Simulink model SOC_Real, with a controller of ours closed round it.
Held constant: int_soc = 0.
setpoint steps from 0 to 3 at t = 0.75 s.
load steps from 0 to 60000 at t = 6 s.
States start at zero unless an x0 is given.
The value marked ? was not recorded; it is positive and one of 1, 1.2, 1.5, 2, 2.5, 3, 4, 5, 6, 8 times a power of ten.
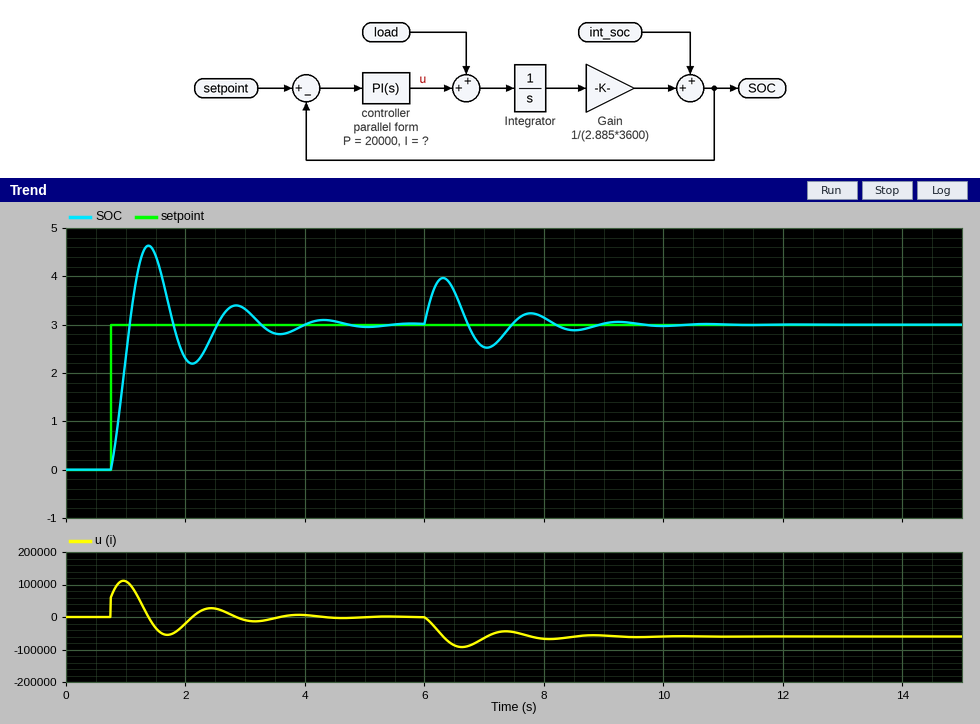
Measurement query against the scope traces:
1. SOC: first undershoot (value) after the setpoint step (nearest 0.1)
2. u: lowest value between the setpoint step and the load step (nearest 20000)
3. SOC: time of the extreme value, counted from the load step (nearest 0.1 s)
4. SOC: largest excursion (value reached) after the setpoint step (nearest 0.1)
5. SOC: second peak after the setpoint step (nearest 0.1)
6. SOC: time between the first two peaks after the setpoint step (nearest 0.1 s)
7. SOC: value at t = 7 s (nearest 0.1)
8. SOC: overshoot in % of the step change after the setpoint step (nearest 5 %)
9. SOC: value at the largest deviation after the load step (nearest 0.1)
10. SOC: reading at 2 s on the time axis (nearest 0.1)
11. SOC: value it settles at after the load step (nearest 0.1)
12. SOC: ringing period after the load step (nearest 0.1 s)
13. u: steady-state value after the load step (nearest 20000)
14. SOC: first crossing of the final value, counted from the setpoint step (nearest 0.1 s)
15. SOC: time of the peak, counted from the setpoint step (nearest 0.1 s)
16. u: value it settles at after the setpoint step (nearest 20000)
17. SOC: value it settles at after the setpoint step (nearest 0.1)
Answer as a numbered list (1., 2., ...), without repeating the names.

1. 2.2
2. -60000
3. 0.3 s
4. 4.6
5. 3.4
6. 1.5 s
7. 2.5
8. 55 %
9. 4.0
10. 2.3
11. 3.0
12. 1.5 s
13. -60000
14. 0.3 s
15. 0.6 s
16. 0
17. 3.0
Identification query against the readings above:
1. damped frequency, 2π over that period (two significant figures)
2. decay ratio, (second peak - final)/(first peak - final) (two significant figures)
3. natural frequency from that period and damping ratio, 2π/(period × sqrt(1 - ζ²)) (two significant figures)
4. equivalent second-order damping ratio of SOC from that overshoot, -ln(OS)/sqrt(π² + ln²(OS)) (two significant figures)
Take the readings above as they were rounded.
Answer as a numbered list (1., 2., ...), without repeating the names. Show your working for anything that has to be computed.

1. 2π / 1.5 = 4.2 rad/s
2. (3.4 - 3) / (4.6 - 3) = 0.25
3. 2π / (1.5 × sqrt(1 - 0.19²)) = 4.3 rad/s
4. ln(0.55) = -0.598; 0.598 / sqrt(9.870 + 0.357) = 0.19
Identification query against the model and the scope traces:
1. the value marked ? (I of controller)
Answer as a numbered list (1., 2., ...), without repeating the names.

1. 200000
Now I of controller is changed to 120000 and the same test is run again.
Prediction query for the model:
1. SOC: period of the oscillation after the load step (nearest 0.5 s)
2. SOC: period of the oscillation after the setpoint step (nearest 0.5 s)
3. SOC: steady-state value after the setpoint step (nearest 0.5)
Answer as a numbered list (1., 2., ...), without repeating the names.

1. 2.0 s
2. 2.0 s
3. 3.0
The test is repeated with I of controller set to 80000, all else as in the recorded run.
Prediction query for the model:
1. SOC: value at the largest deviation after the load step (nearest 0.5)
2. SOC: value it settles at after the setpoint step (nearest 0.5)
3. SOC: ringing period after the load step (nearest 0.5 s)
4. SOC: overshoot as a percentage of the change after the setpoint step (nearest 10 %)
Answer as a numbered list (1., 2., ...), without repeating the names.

1. 4.5
2. 3.0
3. 2.5 s
4. 40 %
